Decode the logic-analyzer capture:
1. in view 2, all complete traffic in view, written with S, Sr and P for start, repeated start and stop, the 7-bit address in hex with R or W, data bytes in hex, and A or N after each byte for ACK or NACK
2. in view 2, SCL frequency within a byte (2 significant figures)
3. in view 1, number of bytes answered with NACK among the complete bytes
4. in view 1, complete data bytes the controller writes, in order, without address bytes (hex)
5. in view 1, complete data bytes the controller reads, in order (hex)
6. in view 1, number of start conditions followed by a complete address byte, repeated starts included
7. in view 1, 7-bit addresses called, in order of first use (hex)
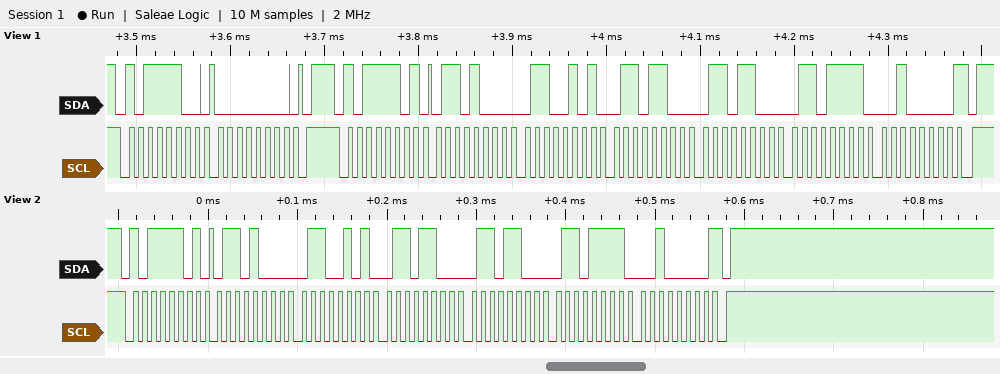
S 5ER A 68 A 65 A 6C A 6C A 6F A 20 N P
100 kHz
1
00
68 65 6C 6C 6F 20
2
0x5E
